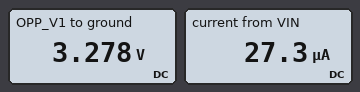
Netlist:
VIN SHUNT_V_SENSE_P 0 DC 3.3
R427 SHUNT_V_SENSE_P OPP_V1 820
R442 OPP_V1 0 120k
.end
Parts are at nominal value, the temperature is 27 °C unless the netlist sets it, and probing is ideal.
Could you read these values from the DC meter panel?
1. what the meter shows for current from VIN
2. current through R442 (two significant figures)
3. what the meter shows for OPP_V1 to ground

27.3 µA
27 µA
3.278 V
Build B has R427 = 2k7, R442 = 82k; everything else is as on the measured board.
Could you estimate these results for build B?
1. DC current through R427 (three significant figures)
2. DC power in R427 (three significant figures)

39.0 µA
4.10 µW
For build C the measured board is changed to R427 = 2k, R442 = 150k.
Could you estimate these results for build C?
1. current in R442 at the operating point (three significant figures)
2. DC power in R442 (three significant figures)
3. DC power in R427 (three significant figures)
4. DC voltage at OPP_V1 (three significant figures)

21.7 µA
70.7 µW
943 nW
3.26 V
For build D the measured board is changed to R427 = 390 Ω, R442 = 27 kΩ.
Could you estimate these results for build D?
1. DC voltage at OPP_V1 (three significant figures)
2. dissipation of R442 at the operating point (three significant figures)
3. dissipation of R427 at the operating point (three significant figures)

3.25 V
392 µW
5.66 µW
